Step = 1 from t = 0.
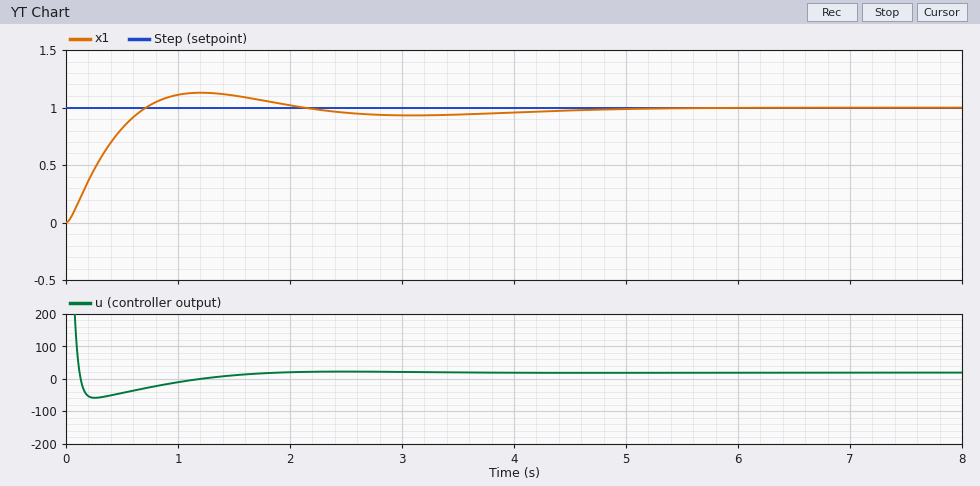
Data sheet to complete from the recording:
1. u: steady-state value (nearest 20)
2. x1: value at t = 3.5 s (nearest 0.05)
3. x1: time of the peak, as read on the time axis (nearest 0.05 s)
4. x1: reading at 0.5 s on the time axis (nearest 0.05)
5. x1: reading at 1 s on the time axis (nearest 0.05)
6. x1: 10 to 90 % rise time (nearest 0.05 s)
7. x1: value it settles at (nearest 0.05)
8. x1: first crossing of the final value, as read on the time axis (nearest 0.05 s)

20
0.95
1.20 s
0.80
1.10
0.50 s
1.00
0.70 s
